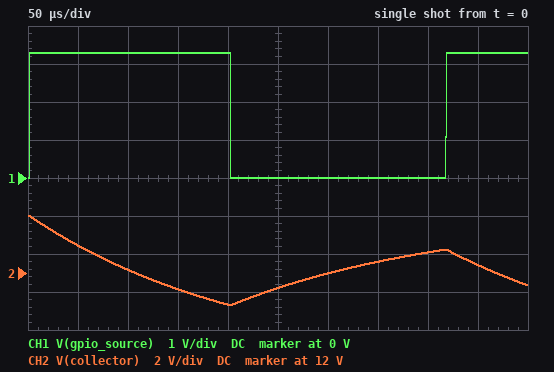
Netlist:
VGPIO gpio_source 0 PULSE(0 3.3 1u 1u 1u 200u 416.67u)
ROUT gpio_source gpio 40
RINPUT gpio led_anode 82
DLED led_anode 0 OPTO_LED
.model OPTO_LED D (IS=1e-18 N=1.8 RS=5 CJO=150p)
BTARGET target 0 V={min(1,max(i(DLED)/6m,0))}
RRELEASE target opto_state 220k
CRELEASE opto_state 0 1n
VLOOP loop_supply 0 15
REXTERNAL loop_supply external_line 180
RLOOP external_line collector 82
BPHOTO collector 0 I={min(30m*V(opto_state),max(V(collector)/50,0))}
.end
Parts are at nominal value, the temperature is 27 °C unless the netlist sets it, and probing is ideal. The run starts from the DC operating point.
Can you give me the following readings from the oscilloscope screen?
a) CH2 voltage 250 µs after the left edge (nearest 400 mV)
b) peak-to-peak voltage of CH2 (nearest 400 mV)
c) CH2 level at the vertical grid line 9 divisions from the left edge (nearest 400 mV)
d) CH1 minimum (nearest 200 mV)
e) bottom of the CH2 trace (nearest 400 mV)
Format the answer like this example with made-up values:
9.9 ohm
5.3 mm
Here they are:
11.2 V
4.8 V
12.4 V
0 V
10.4 V
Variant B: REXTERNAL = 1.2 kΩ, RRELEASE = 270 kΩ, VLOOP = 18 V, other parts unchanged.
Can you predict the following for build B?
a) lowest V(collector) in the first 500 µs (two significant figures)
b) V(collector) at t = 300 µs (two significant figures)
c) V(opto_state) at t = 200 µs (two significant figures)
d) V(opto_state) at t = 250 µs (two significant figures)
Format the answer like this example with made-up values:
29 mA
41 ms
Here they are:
680 mV
3.9 V
520 mV
440 mV
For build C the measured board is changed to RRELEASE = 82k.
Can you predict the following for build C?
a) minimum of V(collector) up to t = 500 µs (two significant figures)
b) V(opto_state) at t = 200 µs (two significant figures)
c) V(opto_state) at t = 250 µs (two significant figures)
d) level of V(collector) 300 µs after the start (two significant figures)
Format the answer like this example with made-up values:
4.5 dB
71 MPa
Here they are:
7.8 V
910 mV
510 mV
13 V
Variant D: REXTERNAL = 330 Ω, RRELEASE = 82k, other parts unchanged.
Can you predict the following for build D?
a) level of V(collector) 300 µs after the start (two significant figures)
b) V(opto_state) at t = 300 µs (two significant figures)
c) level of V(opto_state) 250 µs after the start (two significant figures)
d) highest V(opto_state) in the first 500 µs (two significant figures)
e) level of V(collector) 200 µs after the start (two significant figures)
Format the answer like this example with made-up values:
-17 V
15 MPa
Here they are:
12 V
280 mV
510 mV
910 mV
3.7 V
